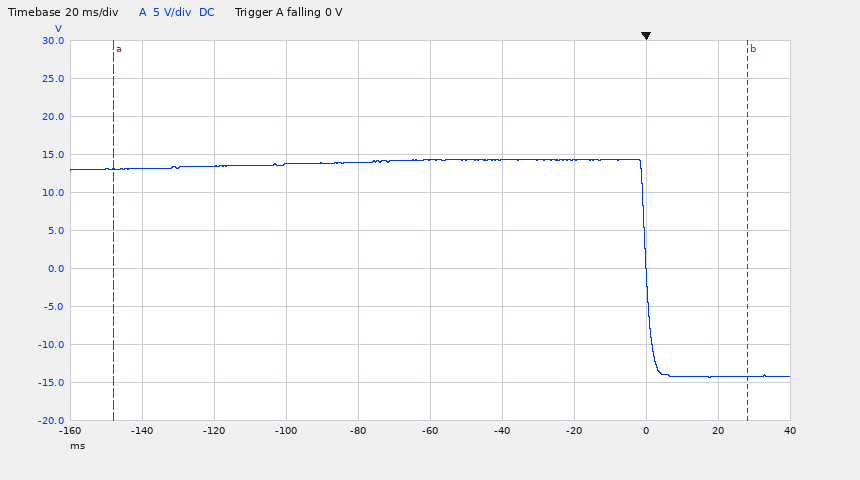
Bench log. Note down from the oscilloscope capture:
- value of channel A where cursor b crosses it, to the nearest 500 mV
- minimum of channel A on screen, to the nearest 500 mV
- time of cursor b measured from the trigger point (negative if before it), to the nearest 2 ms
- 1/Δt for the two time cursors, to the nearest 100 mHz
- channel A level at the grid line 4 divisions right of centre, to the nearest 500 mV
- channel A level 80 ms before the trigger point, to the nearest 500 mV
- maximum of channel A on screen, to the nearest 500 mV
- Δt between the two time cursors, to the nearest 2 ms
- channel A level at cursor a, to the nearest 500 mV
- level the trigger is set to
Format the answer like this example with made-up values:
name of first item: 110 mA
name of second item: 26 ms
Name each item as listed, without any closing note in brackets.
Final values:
value of channel A where cursor b crosses it, to the nearest 500 mV: -14.0 V
minimum of channel A on screen, to the nearest 500 mV: -14.5 V
time of cursor b measured from the trigger point (negative if before it), to the nearest 2 ms: +28 ms
1/Δt for the two time cursors, to the nearest 100 mHz: 5.7 Hz
channel A level at the grid line 4 divisions right of centre, to the nearest 500 mV: -14.0 V
channel A level 80 ms before the trigger point, to the nearest 500 mV: 14.0 V
maximum of channel A on screen, to the nearest 500 mV: 14.5 V
Δt between the two time cursors, to the nearest 2 ms: 176 ms
channel A level at cursor a, to the nearest 500 mV: 13.0 V
level the trigger is set to: 0 V
